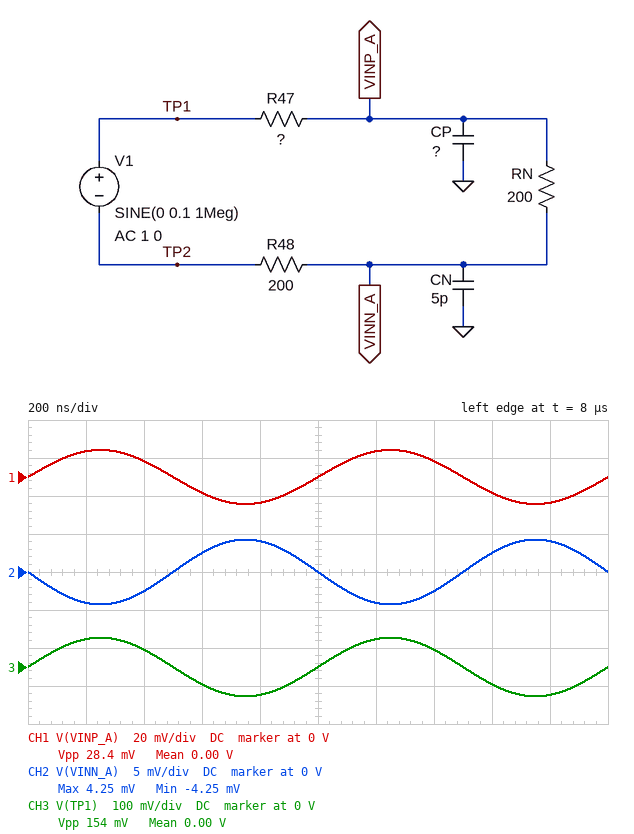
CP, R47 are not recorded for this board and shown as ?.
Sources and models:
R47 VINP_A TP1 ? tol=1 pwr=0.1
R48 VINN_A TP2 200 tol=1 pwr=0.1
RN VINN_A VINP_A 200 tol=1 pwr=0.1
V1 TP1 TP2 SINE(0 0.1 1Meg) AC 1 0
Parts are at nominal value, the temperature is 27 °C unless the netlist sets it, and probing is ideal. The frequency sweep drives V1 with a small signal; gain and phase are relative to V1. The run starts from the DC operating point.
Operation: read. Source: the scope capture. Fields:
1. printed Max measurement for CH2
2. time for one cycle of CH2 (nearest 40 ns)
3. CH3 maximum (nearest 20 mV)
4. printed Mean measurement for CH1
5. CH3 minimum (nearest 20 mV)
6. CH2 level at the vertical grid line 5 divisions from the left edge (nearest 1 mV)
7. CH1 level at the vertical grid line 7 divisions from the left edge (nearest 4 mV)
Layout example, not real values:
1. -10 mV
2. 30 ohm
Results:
1. 4.25 mV
2. 1.00 µs
3. 80 mV
4. 0.00 V
5. -80 mV
6. 0 V
7. 8 mV
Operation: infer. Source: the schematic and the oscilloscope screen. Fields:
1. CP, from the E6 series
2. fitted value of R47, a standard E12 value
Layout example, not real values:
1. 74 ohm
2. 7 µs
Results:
1. 1.5 pF
2. 680 Ω
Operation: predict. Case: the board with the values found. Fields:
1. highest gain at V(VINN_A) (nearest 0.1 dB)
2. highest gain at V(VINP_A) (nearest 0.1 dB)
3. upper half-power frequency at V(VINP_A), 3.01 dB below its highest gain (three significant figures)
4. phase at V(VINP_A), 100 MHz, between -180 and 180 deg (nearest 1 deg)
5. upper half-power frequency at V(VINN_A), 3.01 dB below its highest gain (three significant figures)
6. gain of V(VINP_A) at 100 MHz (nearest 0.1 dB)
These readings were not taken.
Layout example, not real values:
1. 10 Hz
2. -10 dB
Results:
1. -27.4 dB
2. -16.9 dB
3. 846 MHz
4. -7 deg
5. 846 MHz
6. -17.0 dB
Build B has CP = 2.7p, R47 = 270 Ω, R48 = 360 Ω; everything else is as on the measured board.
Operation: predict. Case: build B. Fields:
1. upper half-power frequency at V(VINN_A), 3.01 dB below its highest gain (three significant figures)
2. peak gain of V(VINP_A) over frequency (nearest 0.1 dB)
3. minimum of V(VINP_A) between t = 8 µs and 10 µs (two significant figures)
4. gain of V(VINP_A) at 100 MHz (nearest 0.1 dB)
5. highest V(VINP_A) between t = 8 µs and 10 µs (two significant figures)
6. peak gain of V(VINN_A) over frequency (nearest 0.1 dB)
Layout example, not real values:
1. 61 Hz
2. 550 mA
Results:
1. 598 MHz
2. -16.1 dB
3. -16 mV
4. -16.2 dB
5. 16 mV
6. -21.5 dB
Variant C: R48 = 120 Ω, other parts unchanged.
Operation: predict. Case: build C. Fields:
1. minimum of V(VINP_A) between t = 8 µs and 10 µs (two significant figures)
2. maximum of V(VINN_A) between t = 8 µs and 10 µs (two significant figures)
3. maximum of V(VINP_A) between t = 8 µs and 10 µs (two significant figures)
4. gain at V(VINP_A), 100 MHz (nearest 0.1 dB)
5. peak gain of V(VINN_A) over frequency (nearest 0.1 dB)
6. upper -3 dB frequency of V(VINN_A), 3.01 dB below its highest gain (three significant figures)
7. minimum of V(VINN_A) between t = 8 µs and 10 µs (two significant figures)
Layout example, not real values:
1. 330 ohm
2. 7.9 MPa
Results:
1. -15 mV
2. 4.6 mV
3. 15 mV
4. -16.3 dB
5. -26.7 dB
6. 862 MHz
7. -4.6 mV
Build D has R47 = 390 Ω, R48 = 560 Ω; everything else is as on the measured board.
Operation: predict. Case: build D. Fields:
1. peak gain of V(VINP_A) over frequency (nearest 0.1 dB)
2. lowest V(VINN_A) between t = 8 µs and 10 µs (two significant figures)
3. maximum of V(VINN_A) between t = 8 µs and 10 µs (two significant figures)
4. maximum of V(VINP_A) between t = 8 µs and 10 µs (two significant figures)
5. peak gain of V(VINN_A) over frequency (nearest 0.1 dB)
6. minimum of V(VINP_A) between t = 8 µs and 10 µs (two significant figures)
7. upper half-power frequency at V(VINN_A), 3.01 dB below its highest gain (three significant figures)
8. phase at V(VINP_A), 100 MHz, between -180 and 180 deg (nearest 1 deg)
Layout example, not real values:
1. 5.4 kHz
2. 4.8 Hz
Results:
1. -17.5 dB
2. -4.0 mV
3. 4.0 mV
4. 13 mV
5. -27.9 dB
6. -13 mV
7. 835 MHz
8. -7 deg
